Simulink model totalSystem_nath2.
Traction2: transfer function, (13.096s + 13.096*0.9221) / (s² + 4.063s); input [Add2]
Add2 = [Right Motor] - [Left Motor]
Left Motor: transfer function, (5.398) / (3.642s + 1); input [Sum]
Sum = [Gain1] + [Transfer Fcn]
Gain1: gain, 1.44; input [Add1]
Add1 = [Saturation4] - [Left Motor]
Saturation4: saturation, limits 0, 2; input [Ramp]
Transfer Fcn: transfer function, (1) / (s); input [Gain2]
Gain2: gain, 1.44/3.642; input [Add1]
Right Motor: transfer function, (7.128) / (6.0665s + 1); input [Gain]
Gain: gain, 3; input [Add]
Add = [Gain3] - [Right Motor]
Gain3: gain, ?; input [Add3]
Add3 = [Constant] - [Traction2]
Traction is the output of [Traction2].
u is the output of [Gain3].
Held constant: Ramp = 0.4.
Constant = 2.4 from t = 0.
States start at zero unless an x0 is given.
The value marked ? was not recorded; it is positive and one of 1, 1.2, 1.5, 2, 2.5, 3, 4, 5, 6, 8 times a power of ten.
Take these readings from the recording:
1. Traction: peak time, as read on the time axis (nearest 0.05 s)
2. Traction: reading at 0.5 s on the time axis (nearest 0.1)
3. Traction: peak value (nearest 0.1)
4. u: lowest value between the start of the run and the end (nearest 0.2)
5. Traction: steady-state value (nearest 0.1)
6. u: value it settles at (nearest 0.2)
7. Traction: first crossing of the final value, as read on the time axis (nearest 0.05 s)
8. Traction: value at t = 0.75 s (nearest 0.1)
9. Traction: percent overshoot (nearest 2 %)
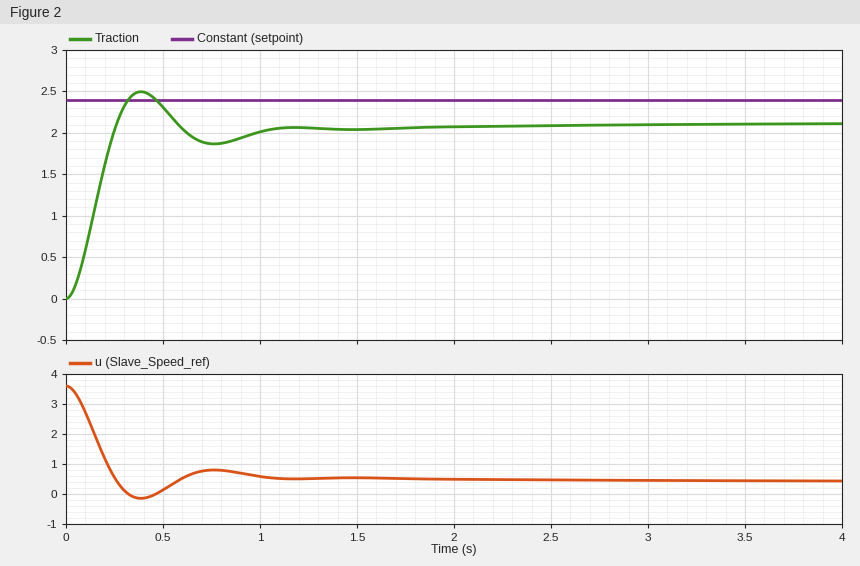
0.40 s
2.3
2.5
-0.2
2.1
0.4
0.25 s
1.9
18 %
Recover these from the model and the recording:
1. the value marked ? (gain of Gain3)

1.5
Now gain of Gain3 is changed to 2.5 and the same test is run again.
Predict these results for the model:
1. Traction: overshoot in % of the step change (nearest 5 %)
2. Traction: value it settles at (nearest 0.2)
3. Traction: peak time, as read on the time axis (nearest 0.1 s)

30 %
2.2
0.3 s
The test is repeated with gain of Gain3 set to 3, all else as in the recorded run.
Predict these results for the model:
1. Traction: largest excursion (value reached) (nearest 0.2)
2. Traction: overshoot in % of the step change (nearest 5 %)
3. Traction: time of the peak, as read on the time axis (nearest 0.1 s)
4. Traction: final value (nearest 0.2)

3.0
35 %
0.3 s
2.2
